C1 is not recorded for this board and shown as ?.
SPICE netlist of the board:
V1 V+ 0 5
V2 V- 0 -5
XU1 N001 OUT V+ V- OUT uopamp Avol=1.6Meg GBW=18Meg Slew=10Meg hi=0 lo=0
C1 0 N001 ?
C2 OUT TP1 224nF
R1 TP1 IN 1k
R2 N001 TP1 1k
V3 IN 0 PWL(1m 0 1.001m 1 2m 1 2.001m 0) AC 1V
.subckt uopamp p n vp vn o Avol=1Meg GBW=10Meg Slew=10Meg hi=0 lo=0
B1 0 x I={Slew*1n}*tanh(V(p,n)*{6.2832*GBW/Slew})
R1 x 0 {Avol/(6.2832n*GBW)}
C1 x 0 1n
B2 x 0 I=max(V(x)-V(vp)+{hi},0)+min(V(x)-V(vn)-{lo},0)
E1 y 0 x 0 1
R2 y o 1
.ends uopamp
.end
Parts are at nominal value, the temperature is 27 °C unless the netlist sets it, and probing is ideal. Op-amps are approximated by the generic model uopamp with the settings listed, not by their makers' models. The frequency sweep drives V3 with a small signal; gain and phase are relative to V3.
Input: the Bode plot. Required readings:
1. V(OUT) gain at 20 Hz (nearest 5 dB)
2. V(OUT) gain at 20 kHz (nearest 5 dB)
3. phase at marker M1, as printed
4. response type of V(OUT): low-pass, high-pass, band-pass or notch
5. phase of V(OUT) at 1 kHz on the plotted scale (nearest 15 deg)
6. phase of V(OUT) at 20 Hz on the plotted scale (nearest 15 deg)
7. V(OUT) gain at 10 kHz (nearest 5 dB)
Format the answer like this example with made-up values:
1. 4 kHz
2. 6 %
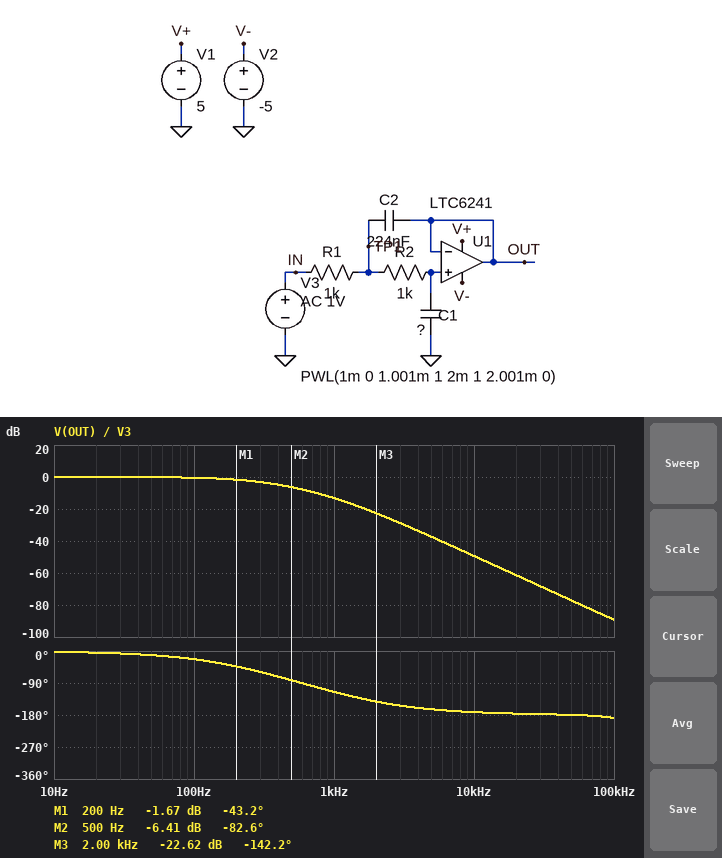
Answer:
1. 0 dB
2. -60 dB
3. -43.2 deg
4. low-pass
5. -120 deg
6. 0 deg
7. -50 dB
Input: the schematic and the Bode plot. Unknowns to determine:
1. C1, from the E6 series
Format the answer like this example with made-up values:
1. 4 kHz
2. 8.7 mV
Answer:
1. 330 nF
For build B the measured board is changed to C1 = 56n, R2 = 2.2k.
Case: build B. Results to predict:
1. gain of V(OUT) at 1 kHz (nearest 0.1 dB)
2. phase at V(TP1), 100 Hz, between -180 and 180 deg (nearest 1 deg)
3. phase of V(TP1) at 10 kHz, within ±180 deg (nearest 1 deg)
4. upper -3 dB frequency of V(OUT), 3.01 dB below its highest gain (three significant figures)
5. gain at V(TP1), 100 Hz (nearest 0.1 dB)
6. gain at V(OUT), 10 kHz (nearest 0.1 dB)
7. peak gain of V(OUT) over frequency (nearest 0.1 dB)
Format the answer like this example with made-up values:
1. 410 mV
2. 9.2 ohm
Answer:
1. -1.1 dB
2. -2 deg
3. -91 deg
4. 1.10 kHz
5. 0.1 dB
6. -40.7 dB
7. 0.8 dB
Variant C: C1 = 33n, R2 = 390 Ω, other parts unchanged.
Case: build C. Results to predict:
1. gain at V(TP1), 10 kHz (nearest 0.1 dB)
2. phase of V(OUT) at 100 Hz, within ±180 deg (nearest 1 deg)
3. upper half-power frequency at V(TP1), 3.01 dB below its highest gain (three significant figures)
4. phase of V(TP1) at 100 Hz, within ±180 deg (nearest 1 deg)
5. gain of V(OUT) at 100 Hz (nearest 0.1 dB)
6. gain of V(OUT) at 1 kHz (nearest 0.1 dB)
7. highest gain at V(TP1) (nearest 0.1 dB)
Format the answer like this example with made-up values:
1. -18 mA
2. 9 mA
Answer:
1. -18.5 dB
2. -2 deg
3. 3.56 kHz
4. -1 deg
5. 0 dB
6. 0.6 dB
7. 2.4 dB
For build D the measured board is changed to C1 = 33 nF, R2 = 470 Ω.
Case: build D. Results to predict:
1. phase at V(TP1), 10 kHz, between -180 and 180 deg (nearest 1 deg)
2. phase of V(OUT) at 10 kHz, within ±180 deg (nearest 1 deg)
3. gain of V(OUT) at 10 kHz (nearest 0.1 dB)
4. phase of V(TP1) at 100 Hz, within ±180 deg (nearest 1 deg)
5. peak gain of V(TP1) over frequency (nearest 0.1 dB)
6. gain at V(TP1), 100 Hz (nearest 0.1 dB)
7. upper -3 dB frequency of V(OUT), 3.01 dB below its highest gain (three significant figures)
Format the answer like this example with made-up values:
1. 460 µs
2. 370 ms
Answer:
1. -122 deg
2. -167 deg
3. -22.3 dB
4. -1 deg
5. 2.7 dB
6. 0 dB
7. 3.21 kHz
